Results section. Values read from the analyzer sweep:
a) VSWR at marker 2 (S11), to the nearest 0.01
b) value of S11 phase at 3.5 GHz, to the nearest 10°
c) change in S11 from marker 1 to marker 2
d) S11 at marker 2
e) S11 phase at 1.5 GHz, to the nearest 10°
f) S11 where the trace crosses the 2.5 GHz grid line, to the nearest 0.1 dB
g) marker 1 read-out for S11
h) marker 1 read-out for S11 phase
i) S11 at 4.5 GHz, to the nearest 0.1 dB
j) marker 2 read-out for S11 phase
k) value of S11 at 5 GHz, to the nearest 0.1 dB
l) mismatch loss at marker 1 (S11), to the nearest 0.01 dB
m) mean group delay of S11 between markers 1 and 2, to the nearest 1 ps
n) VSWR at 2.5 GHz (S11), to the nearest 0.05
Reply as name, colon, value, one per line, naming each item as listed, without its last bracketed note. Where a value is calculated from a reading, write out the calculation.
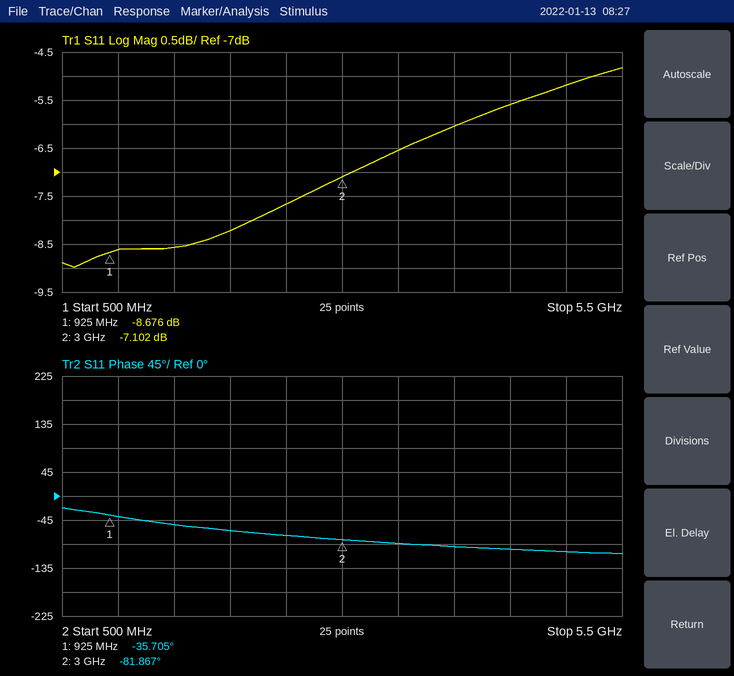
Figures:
VSWR at marker 2 (S11), to the nearest 0.01: (1 + 0.4415)/(1 − 0.4415) ≈ 2.58
value of S11 phase at 3.5 GHz, to the nearest 10°: -90°
change in S11 from marker 1 to marker 2: -7.102 − (-8.676) = 1.574 dB
S11 at marker 2: -7.102 dB
S11 phase at 1.5 GHz, to the nearest 10°: -50°
S11 where the trace crosses the 2.5 GHz grid line, to the nearest 0.1 dB: -7.7 dB
marker 1 read-out for S11: -8.676 dB
marker 1 read-out for S11 phase: -35.705°
S11 at 4.5 GHz, to the nearest 0.1 dB: -5.6 dB
marker 2 read-out for S11 phase: -81.867°
value of S11 at 5 GHz, to the nearest 0.1 dB: -5.2 dB
mismatch loss at marker 1 (S11), to the nearest 0.01 dB: −10 log10(1 − 10^(-8.676/10)) ≈ 0.63 dB
mean group delay of S11 between markers 1 and 2, to the nearest 1 ps: −(-81.867° − (-35.705°))/(360° × 2.075 GHz) ≈ 62 ps
VSWR at 2.5 GHz (S11), to the nearest 0.05: |Γ| = 10^(-7.7/20) = 0.4121; VSWR = (1 + 0.4121)/(1 − 0.4121) ≈ 2.40
